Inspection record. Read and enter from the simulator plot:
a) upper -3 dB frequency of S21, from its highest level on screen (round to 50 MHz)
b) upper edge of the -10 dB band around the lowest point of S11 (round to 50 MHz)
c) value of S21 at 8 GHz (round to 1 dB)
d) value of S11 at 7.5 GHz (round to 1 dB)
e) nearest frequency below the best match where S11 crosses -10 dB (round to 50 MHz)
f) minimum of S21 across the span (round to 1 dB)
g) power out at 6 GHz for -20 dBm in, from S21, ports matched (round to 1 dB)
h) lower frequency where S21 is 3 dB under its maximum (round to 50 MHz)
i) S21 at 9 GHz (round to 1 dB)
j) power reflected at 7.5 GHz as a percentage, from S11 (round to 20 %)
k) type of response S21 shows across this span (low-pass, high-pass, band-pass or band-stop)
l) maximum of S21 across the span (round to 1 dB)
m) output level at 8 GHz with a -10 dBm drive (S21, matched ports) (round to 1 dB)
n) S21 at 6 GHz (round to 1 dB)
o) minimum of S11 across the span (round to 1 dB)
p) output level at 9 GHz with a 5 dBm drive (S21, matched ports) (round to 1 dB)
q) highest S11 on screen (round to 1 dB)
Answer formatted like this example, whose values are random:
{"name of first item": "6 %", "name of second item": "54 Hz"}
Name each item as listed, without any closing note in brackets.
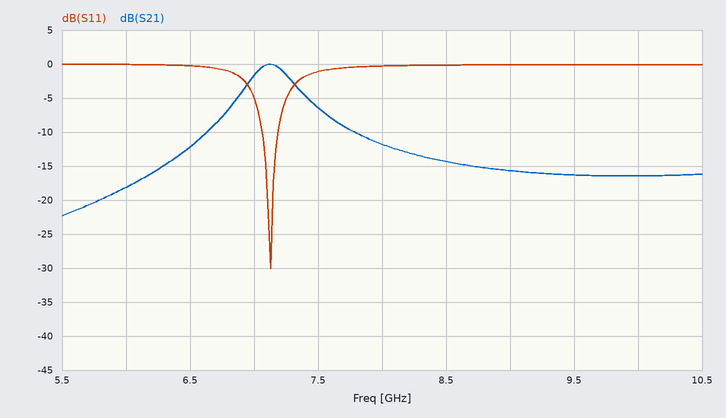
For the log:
{"upper -3 dB frequency of S21, from its highest level on screen": "7.30 GHz", "upper edge of the -10 dB band around the lowest point of S11": "7.20 GHz", "value of S21 at 8 GHz": "-12 dB", "value of S11 at 7.5 GHz": "-1 dB", "nearest frequency below the best match where S11 crosses -10 dB": "7.05 GHz", "minimum of S21 across the span": "-22 dB", "power out at 6 GHz for -20 dBm in, from S21, ports matched": "-38 dBm", "lower frequency where S21 is 3 dB under its maximum": "6.95 GHz", "S21 at 9 GHz": "-16 dB", "power reflected at 7.5 GHz as a percentage, from S11": "80 %", "type of response S21 shows across this span": "band-pass", "maximum of S21 across the span": "0 dB", "output level at 8 GHz with a -10 dBm drive (S21, matched ports)": "-22 dBm", "S21 at 6 GHz": "-18 dB", "minimum of S11 across the span": "-30 dB", "output level at 9 GHz with a 5 dBm drive (S21, matched ports)": "-11 dBm", "highest S11 on screen": "0 dB"}
